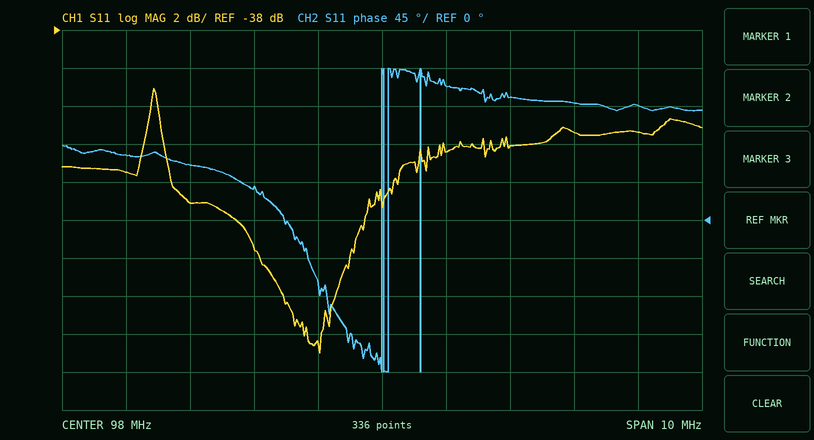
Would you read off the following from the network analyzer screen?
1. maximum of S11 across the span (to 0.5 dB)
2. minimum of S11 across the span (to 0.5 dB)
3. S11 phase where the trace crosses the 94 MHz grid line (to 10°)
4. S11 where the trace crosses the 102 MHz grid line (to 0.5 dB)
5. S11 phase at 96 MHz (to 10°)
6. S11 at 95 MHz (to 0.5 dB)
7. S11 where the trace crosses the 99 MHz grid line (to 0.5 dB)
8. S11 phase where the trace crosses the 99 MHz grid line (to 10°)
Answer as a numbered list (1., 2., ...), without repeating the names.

1. -41.0 dB
2. -55.0 dB
3. 80°
4. -43.5 dB
5. 40°
6. -47.0 dB
7. -44.5 dB
8. 160°
